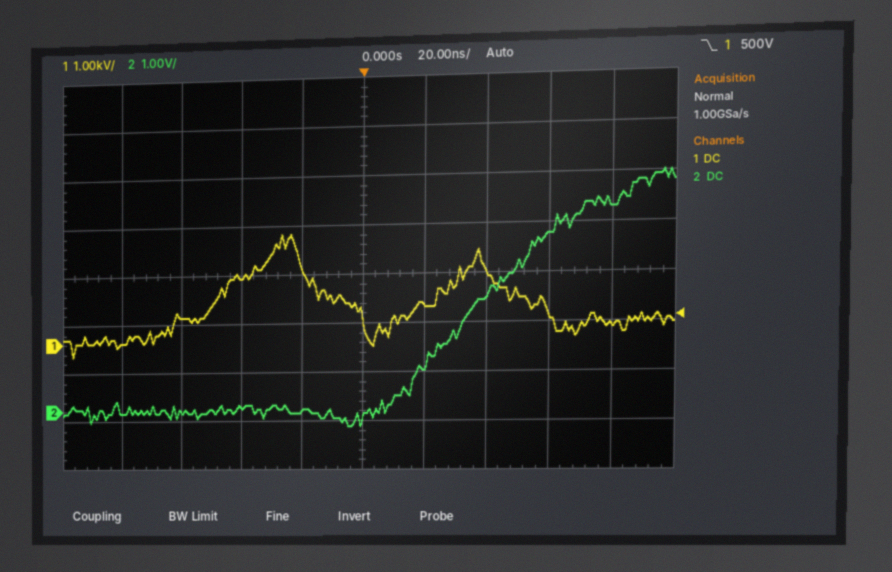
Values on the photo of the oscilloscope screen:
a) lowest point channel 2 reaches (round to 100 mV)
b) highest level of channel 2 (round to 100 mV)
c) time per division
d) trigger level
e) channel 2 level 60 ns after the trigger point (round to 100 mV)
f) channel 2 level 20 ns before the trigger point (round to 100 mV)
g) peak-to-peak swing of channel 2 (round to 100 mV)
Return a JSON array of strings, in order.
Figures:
["-300 mV", "4.8 V", "20 ns", "500 V", "3.6 V", "0.0 V", "5.1 V"]
